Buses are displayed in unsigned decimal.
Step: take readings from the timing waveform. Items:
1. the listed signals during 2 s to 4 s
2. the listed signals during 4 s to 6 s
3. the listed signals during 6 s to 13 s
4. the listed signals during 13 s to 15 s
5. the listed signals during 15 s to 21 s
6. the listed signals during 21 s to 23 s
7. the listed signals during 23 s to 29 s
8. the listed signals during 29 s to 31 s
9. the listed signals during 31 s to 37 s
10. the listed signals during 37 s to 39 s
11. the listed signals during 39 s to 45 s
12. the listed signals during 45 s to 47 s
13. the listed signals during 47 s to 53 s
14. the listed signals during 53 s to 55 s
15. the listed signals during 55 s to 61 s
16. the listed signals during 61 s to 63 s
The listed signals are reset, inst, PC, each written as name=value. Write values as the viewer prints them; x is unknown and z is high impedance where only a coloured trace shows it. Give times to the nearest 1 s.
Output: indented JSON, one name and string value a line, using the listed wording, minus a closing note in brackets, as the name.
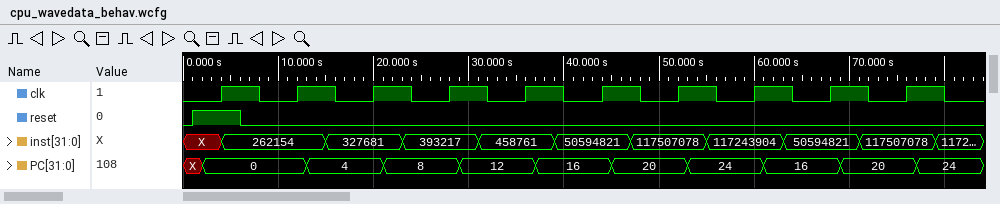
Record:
{
  "the listed signals during 2 s to 4 s": "reset=1, inst=X, PC=0",
  "the listed signals during 4 s to 6 s": "reset=1, inst=262154, PC=0",
  "the listed signals during 6 s to 13 s": "reset=0, inst=262154, PC=0",
  "the listed signals during 13 s to 15 s": "reset=0, inst=262154, PC=4",
  "the listed signals during 15 s to 21 s": "reset=0, inst=327681, PC=4",
  "the listed signals during 21 s to 23 s": "reset=0, inst=327681, PC=8",
  "the listed signals during 23 s to 29 s": "reset=0, inst=393217, PC=8",
  "the listed signals during 29 s to 31 s": "reset=0, inst=393217, PC=12",
  "the listed signals during 31 s to 37 s": "reset=0, inst=458761, PC=12",
  "the listed signals during 37 s to 39 s": "reset=0, inst=458761, PC=16",
  "the listed signals during 39 s to 45 s": "reset=0, inst=50594821, PC=16",
  "the listed signals during 45 s to 47 s": "reset=0, inst=50594821, PC=20",
  "the listed signals during 47 s to 53 s": "reset=0, inst=117507078, PC=20",
  "the listed signals during 53 s to 55 s": "reset=0, inst=117507078, PC=24",
  "the listed signals during 55 s to 61 s": "reset=0, inst=117243904, PC=24",
  "the listed signals during 61 s to 63 s": "reset=0, inst=117243904, PC=16"
}
